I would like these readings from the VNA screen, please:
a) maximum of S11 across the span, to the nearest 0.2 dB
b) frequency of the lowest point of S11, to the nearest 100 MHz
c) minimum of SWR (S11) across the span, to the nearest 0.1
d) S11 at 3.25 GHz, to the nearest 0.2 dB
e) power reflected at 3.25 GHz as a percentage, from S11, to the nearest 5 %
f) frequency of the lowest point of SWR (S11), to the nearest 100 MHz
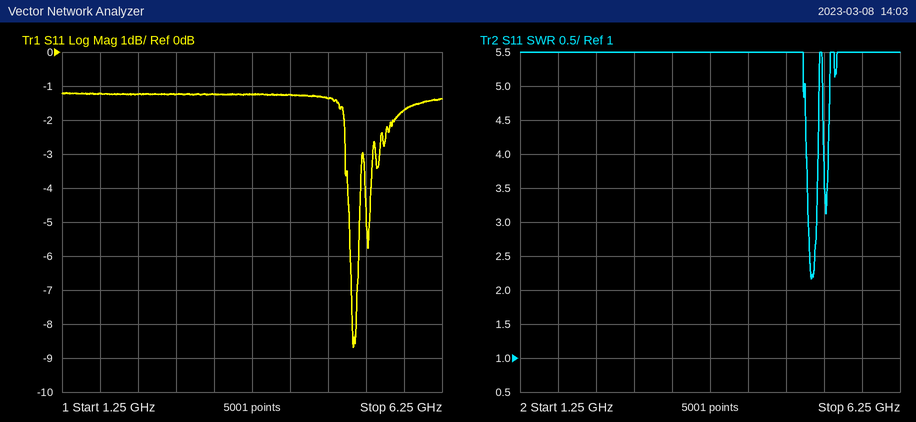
-1.2 dB
5.1 GHz
2.2
-1.2 dB
75 %
5.1 GHz
